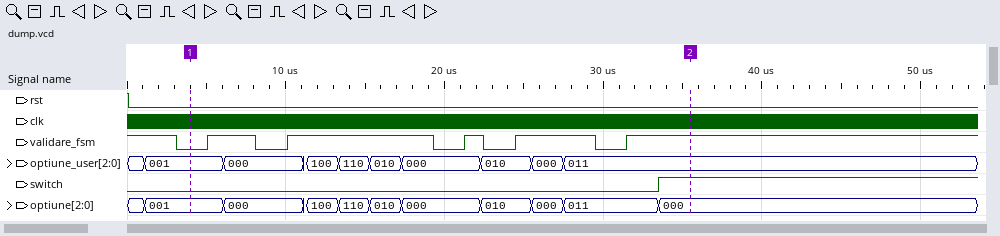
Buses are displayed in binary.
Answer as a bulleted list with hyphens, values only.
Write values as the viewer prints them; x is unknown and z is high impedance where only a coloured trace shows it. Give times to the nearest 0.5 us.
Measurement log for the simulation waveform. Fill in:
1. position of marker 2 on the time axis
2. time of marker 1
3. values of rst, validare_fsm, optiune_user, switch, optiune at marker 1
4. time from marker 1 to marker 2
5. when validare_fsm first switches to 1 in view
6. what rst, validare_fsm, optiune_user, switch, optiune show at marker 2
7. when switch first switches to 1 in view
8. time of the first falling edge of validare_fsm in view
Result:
- 35.5 us
- 4 us
- rst=0, validare_fsm=0, optiune_user=001, switch=0, optiune=001
- 31.5 us
- 5 us
- rst=0, validare_fsm=1, optiune_user=011, switch=1, optiune=000
- 33.5 us
- 3 us
